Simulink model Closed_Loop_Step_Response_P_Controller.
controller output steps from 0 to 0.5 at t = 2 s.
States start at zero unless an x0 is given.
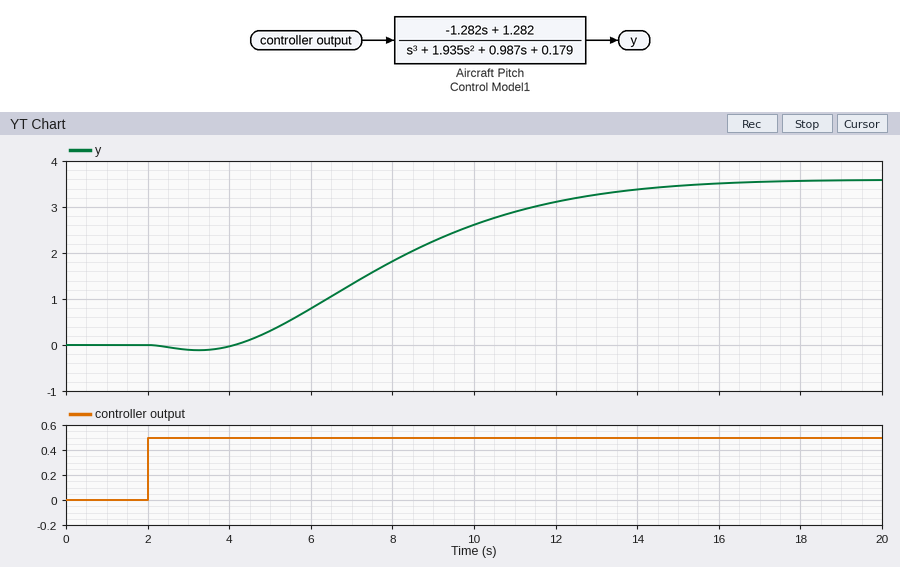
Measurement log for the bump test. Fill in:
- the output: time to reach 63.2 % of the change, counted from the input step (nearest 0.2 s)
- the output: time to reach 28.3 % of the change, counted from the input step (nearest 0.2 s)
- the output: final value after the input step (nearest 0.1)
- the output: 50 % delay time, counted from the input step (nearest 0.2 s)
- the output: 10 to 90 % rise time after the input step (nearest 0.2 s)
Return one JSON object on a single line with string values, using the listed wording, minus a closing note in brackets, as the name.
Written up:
{"the output: time to reach 63.2 % of the change, counted from the input step": "7.0 s", "the output: time to reach 28.3 % of the change, counted from the input step": "4.4 s", "the output: final value after the input step": "3.6", "the output: 50 % delay time, counted from the input step": "6.0 s", "the output: 10 to 90 % rise time after the input step": "7.6 s"}
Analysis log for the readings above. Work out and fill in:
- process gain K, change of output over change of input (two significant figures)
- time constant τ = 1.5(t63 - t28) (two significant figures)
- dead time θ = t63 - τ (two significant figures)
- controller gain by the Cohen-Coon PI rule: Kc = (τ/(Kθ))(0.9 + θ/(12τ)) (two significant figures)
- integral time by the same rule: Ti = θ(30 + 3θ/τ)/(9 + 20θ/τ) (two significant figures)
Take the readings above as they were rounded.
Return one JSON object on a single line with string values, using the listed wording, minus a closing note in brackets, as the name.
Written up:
{"process gain K, change of output over change of input": "7.2", "time constant τ = 1.5(t63 - t28)": "3.9 s", "dead time θ = t63 - τ": "3.1 s", "controller gain by the Cohen-Coon PI rule: Kc = (τ/(Kθ))(0.9 + θ/(12τ))": "0.17", "integral time by the same rule: Ti = θ(30 + 3θ/τ)/(9 + 20θ/τ)": "4.0 s"}
